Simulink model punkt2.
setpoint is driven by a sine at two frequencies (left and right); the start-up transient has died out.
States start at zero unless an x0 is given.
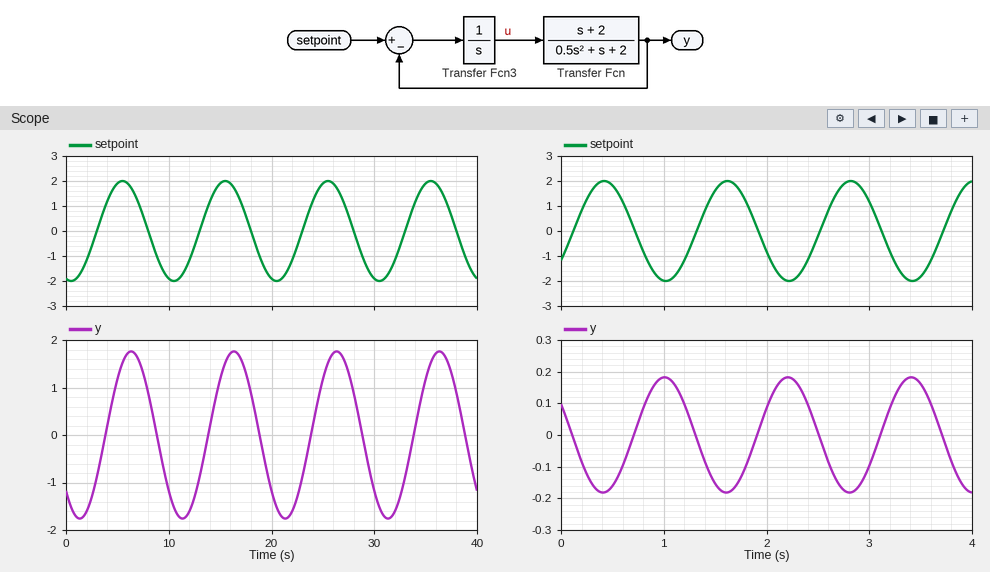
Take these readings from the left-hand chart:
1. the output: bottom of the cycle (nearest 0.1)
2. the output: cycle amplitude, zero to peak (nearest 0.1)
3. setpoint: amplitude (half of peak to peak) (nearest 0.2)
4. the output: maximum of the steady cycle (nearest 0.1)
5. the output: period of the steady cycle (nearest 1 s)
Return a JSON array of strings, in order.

["-1.8", "1.8", "2.0", "1.8", "10 s"]
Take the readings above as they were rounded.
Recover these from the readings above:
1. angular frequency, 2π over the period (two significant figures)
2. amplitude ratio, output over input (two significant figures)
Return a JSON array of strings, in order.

["0.63 rad/s", "0.90"]
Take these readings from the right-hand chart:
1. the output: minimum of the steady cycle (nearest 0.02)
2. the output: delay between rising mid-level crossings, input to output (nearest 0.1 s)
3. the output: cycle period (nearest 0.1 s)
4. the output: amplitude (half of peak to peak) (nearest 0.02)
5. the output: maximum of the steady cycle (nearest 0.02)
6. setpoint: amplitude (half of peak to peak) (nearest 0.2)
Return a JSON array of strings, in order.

["-0.18", "0.6 s", "1.2 s", "0.18", "0.18", "2.0"]
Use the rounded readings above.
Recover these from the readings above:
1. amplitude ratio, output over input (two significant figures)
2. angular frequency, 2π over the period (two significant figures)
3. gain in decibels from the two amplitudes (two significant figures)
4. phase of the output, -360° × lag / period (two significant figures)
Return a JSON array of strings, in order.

["0.090", "5.2 rad/s", "-21 dB", "-180°"]
